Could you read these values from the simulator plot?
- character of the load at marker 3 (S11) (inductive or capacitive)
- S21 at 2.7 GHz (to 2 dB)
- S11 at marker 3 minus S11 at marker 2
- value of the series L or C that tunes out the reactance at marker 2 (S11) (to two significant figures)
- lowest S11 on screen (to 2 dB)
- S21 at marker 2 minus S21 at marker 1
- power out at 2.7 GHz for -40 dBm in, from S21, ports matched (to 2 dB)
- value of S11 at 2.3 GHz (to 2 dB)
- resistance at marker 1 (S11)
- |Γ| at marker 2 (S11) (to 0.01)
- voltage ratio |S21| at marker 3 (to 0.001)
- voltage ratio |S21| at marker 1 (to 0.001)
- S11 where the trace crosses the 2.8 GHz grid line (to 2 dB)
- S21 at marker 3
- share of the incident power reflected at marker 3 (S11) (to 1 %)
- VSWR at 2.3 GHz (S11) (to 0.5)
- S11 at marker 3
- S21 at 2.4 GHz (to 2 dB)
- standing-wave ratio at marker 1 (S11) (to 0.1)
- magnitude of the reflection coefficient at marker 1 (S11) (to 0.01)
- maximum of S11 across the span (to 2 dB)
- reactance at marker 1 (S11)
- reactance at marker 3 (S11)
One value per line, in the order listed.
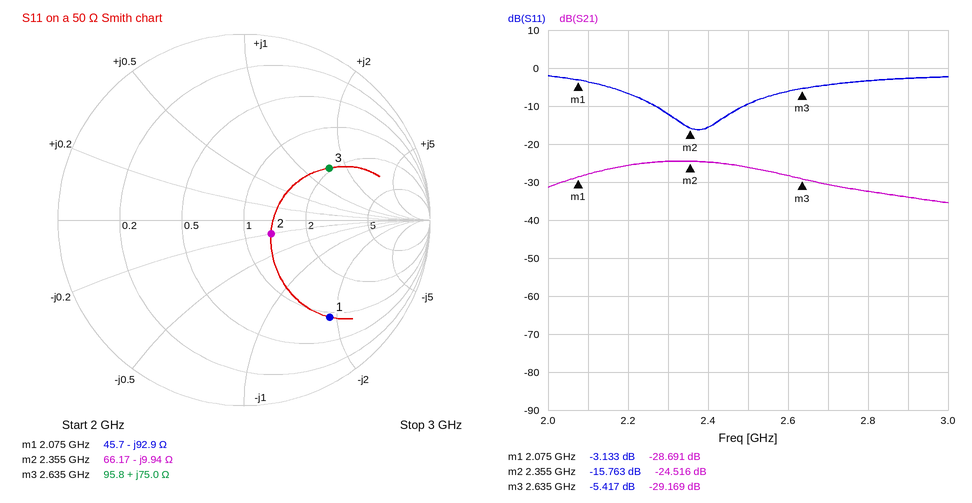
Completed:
inductive
-30 dB
10.346 dB
670 pH
-16 dB
4.175 dB
-70 dBm
-12 dB
45.7 Ω
0.16
0.035
0.037
-4 dB
-29.169 dB
29 %
1.5
-5.417 dB
-24 dB
5.6
0.70
-2 dB
-92.9 Ω
+75.0 Ω
